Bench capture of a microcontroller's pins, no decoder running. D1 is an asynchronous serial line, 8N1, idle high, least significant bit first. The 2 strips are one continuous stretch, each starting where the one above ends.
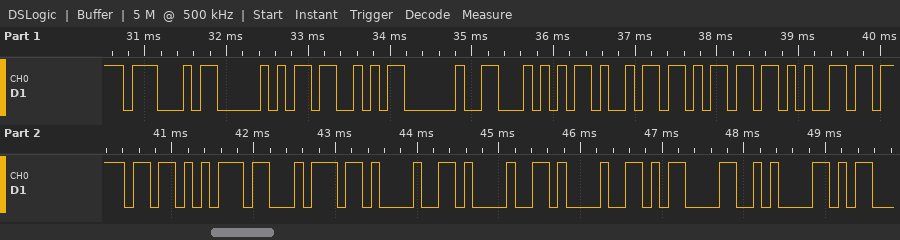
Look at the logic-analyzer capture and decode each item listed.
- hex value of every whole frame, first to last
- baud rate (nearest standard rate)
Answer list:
47 50 53 20 54 69 6D 65 6F 75 74 21 21 21 0D 0A
9600 baud
